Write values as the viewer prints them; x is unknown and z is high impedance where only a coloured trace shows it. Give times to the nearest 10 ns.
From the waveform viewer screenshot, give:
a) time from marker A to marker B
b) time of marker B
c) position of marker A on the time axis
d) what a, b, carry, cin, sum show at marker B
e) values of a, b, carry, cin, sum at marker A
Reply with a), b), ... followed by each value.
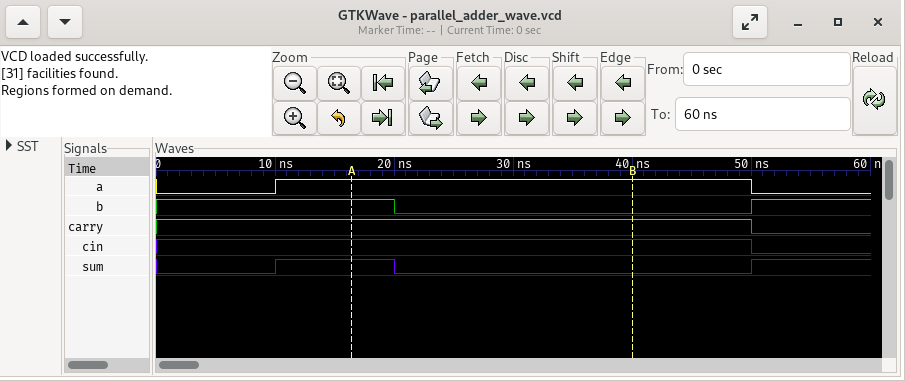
a) 20 ns
b) 40 ns
c) 20 ns
d) a=1, b=0, carry=1, cin=1, sum=0
e) a=1, b=1, carry=1, cin=1, sum=1
